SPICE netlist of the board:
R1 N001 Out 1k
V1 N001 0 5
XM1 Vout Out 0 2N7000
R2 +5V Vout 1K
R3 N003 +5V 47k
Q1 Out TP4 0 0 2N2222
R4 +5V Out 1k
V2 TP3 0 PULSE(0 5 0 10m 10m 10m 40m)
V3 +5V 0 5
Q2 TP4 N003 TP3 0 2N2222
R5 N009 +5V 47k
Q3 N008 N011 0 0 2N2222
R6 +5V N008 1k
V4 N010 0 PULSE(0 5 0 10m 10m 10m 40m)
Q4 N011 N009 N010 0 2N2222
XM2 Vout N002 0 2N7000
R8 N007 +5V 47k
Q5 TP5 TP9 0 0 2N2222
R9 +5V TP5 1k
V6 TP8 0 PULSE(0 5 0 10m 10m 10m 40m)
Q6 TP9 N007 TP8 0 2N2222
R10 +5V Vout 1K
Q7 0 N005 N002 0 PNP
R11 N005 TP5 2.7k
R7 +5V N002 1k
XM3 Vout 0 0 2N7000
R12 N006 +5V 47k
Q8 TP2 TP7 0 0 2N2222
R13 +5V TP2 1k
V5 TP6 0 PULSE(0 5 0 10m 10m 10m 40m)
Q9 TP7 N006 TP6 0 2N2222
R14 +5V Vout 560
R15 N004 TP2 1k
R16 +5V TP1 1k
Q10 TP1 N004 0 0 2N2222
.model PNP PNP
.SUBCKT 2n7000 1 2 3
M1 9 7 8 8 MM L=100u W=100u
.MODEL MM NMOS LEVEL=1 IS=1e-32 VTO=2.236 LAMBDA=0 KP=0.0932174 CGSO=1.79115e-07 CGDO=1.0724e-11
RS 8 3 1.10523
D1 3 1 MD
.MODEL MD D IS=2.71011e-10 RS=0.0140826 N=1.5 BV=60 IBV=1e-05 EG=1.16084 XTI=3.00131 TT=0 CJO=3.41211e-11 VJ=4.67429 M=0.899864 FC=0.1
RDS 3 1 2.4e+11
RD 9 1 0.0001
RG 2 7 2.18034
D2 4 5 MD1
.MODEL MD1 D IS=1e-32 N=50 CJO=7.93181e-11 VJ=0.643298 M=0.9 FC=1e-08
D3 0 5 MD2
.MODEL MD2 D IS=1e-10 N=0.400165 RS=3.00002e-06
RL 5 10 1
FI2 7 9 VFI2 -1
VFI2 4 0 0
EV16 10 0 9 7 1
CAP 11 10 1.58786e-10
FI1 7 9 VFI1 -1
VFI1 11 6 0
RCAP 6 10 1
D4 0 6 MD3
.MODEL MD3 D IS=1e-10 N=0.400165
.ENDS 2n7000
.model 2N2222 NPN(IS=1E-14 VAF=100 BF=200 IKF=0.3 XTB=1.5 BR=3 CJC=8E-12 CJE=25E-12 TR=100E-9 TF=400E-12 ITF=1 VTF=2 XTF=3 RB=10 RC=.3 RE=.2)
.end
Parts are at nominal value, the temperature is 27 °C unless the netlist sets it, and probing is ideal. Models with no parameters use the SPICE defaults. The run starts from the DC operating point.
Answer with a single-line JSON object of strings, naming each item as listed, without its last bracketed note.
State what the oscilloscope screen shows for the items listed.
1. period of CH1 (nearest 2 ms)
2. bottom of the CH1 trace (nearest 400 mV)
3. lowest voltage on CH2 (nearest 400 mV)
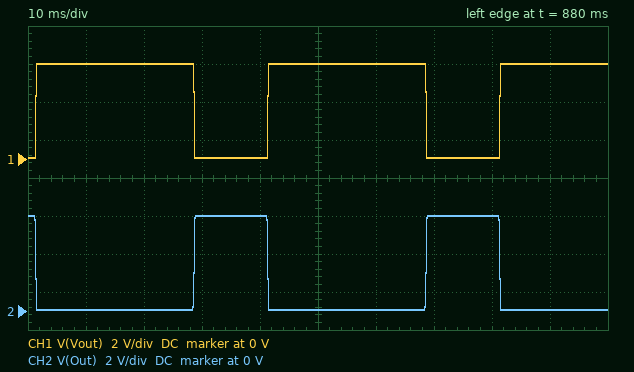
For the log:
{"period of CH1": "40 ms", "bottom of the CH1 trace": "0 V", "lowest voltage on CH2": "0 V"}
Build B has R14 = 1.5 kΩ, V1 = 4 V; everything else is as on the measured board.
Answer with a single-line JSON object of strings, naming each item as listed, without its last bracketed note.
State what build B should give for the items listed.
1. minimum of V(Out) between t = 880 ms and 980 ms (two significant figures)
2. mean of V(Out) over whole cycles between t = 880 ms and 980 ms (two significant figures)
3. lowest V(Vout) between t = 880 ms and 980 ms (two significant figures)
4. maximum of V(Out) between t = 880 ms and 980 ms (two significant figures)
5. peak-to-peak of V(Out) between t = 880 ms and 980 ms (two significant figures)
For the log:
{"minimum of V(Out) between t = 880 ms and 980 ms": "71 mV", "mean of V(Out) over whole cycles between t = 880 ms and 980 ms": "1.5 V", "lowest V(Vout) between t = 880 ms and 980 ms": "36 mV", "maximum of V(Out) between t = 880 ms and 980 ms": "4.5 V", "peak-to-peak of V(Out) between t = 880 ms and 980 ms": "4.4 V"}
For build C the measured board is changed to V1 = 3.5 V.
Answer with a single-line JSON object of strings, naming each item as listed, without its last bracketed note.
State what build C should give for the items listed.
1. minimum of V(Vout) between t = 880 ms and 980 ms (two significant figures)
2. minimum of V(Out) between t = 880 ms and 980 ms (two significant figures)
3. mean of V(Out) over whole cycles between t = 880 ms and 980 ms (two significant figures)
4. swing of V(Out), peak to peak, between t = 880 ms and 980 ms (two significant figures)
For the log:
{"minimum of V(Vout) between t = 880 ms and 980 ms": "53 mV", "minimum of V(Out) between t = 880 ms and 980 ms": "69 mV", "mean of V(Out) over whole cycles between t = 880 ms and 980 ms": "1.4 V", "swing of V(Out), peak to peak, between t = 880 ms and 980 ms": "4.2 V"}
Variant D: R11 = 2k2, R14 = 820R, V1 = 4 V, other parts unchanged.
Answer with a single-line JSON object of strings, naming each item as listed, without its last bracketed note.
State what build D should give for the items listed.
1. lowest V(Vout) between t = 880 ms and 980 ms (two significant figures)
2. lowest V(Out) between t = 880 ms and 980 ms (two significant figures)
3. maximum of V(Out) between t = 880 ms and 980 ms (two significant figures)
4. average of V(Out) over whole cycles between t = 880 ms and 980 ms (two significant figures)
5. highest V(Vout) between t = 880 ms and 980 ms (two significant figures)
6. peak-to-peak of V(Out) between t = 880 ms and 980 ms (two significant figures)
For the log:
{"lowest V(Vout) between t = 880 ms and 980 ms": "43 mV", "lowest V(Out) between t = 880 ms and 980 ms": "71 mV", "maximum of V(Out) between t = 880 ms and 980 ms": "4.5 V", "average of V(Out) over whole cycles between t = 880 ms and 980 ms": "1.5 V", "highest V(Vout) between t = 880 ms and 980 ms": "5.0 V", "peak-to-peak of V(Out) between t = 880 ms and 980 ms": "4.4 V"}
